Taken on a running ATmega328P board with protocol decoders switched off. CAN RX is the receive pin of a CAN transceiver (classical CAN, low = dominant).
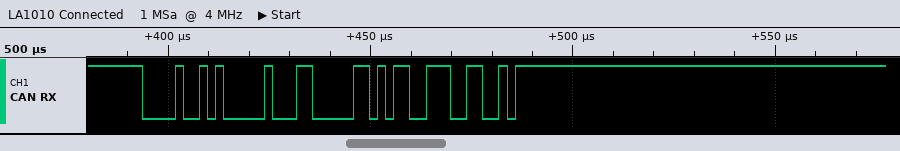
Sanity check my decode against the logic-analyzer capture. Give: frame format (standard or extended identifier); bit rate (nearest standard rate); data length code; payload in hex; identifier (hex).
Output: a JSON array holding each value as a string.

["standard", "500 kbit/s", "1", "82", "0x094"]
